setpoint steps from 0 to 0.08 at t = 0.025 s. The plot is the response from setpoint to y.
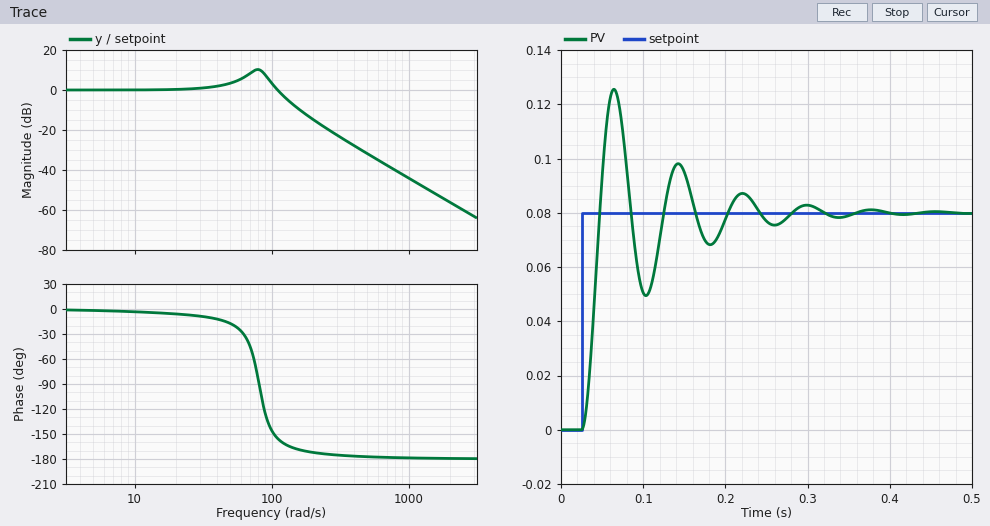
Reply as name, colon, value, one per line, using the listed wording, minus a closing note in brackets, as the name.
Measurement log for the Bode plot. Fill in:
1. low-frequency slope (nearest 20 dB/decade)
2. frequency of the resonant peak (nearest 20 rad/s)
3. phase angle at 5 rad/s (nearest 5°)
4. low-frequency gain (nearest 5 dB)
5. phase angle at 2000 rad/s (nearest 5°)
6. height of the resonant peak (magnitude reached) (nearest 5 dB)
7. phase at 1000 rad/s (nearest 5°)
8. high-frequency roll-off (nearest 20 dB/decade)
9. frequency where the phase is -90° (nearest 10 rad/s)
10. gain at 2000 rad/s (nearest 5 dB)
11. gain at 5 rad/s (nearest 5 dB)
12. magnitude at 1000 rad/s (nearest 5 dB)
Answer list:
low-frequency slope: 0 dB/decade
frequency of the resonant peak: 80 rad/s
phase angle at 5 rad/s: 0°
low-frequency gain: 0 dB
phase angle at 2000 rad/s: -180°
height of the resonant peak (magnitude reached): 10 dB
phase at 1000 rad/s: -180°
high-frequency roll-off: -40 dB/decade
frequency where the phase is -90°: 80 rad/s
gain at 2000 rad/s: -55 dB
gain at 5 rad/s: 0 dB
magnitude at 1000 rad/s: -45 dB
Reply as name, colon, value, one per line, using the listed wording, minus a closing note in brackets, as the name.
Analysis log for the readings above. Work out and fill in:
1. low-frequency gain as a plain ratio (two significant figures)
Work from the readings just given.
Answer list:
low-frequency gain as a plain ratio: 1.0
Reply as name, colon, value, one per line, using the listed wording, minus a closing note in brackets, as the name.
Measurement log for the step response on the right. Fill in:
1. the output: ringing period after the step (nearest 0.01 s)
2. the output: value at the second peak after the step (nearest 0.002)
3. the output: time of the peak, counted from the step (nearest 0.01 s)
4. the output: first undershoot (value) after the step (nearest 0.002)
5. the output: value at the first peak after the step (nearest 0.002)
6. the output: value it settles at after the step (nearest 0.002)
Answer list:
the output: ringing period after the step: 0.08 s
the output: value at the second peak after the step: 0.098
the output: time of the peak, counted from the step: 0.04 s
the output: first undershoot (value) after the step: 0.050
the output: value at the first peak after the step: 0.126
the output: value it settles at after the step: 0.080
